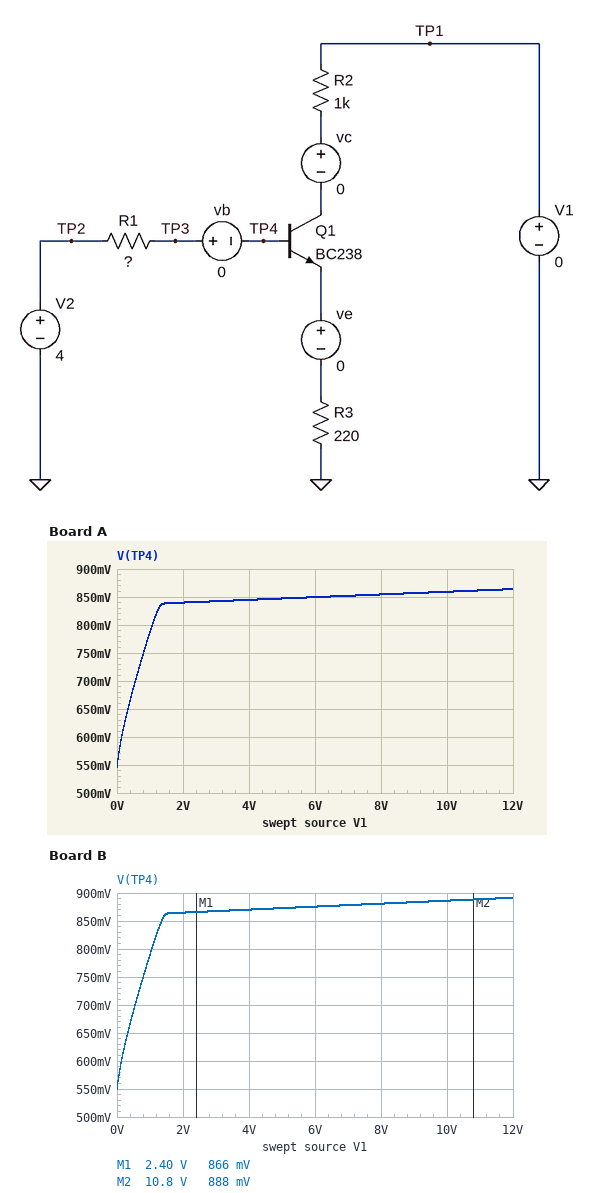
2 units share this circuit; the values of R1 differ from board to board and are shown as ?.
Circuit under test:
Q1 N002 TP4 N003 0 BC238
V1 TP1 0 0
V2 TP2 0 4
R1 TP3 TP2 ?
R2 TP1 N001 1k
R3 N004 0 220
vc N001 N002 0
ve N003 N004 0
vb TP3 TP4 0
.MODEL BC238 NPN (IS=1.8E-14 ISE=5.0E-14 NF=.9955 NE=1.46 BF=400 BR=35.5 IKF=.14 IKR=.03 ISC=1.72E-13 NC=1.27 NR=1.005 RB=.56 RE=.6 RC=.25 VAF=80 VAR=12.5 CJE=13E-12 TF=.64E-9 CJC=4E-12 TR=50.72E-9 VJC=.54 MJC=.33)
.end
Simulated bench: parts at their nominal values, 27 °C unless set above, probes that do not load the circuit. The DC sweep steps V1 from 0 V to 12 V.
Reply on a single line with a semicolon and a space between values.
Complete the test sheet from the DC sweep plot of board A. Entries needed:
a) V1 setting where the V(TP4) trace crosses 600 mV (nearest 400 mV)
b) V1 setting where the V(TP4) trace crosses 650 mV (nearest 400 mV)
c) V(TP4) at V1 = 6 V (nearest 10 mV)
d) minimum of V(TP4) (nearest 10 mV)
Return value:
0 V; 400 mV; 850 mV; 550 mV
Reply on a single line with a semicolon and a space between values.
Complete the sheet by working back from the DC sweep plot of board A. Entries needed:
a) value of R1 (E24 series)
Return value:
910 kΩ
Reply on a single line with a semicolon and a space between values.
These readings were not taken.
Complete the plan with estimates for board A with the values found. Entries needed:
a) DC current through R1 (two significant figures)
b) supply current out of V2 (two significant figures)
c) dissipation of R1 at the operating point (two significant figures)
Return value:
3.8 µA; 3.8 µA; 13 µW
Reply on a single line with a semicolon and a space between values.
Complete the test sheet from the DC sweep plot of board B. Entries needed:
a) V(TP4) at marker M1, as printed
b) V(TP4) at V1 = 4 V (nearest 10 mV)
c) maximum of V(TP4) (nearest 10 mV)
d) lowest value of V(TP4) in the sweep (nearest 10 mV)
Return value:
866 mV; 870 mV; 890 mV; 550 mV
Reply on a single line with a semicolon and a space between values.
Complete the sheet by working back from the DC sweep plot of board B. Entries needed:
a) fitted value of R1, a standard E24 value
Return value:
820 kΩ
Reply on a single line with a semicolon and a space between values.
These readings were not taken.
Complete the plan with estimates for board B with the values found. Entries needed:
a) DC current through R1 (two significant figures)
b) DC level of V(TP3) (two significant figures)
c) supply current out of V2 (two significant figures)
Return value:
4.2 µA; 550 mV; 4.2 µA
